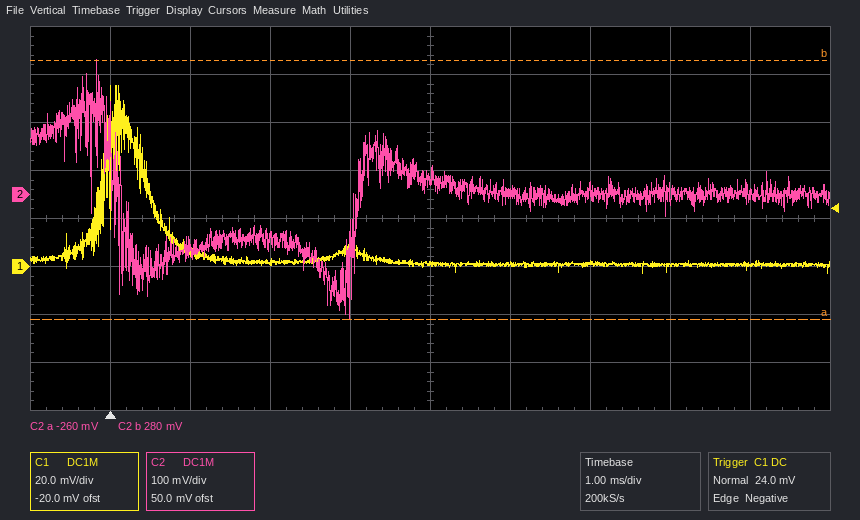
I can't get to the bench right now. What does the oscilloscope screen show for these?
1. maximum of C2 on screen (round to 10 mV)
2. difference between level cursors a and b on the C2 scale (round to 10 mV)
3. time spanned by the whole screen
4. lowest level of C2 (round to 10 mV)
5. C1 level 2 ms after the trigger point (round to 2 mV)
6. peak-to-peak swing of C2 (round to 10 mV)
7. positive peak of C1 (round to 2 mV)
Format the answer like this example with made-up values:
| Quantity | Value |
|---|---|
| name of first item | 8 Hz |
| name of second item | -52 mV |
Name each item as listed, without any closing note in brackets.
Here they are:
| Quantity | Value |
|---|---|
| maximum of C2 on screen | 280 mV |
| difference between level cursors a and b on the C2 scale | 540 mV |
| time spanned by the whole screen | 10 ms |
| lowest level of C2 | -260 mV |
| C1 level 2 ms after the trigger point | 2 mV |
| peak-to-peak swing of C2 | 540 mV |
| positive peak of C1 | 76 mV |
